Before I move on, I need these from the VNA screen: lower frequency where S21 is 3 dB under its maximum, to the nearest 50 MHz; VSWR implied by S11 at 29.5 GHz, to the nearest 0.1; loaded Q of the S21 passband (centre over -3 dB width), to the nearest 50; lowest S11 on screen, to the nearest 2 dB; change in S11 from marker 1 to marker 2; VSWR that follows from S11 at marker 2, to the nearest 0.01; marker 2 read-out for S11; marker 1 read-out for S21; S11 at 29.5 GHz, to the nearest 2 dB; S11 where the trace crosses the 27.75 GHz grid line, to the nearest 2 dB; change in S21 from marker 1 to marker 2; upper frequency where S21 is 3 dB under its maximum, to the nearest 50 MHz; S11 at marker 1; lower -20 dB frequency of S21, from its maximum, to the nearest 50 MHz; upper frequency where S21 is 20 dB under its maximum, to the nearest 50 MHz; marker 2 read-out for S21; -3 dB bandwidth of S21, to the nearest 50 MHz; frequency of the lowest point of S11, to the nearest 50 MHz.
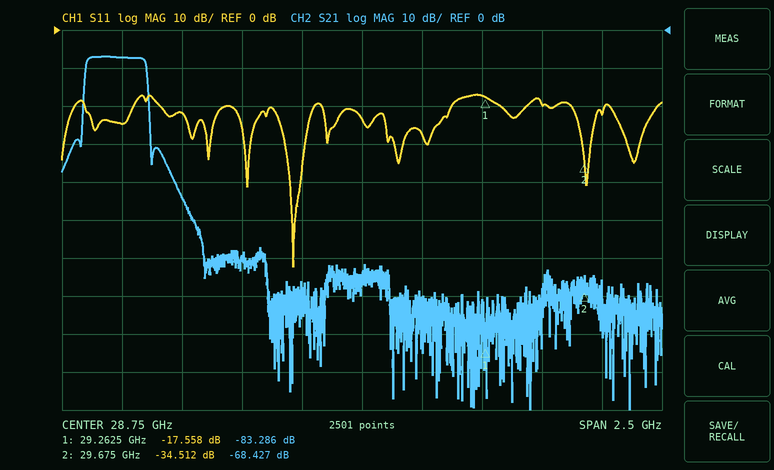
27.60 GHz
1.2
100
-62 dB
-16.954 dB
1.04
-34.512 dB
-83.286 dB
-20 dB
-24 dB
14.859 dB
27.85 GHz
-17.558 dB
27.60 GHz
27.85 GHz
-68.427 dB
250 MHz
28.45 GHz
